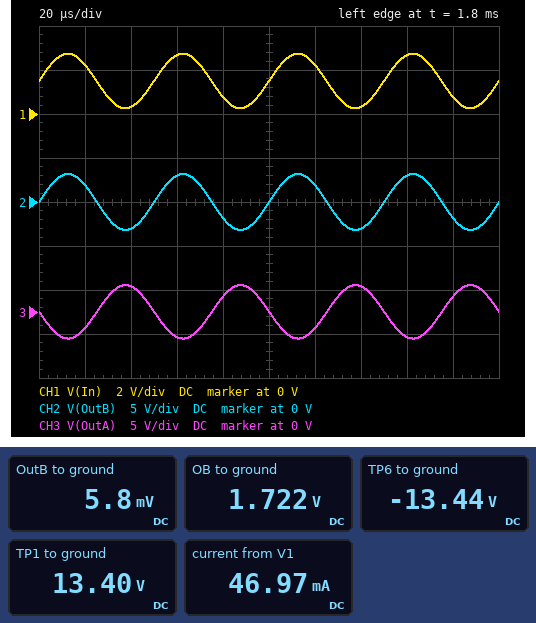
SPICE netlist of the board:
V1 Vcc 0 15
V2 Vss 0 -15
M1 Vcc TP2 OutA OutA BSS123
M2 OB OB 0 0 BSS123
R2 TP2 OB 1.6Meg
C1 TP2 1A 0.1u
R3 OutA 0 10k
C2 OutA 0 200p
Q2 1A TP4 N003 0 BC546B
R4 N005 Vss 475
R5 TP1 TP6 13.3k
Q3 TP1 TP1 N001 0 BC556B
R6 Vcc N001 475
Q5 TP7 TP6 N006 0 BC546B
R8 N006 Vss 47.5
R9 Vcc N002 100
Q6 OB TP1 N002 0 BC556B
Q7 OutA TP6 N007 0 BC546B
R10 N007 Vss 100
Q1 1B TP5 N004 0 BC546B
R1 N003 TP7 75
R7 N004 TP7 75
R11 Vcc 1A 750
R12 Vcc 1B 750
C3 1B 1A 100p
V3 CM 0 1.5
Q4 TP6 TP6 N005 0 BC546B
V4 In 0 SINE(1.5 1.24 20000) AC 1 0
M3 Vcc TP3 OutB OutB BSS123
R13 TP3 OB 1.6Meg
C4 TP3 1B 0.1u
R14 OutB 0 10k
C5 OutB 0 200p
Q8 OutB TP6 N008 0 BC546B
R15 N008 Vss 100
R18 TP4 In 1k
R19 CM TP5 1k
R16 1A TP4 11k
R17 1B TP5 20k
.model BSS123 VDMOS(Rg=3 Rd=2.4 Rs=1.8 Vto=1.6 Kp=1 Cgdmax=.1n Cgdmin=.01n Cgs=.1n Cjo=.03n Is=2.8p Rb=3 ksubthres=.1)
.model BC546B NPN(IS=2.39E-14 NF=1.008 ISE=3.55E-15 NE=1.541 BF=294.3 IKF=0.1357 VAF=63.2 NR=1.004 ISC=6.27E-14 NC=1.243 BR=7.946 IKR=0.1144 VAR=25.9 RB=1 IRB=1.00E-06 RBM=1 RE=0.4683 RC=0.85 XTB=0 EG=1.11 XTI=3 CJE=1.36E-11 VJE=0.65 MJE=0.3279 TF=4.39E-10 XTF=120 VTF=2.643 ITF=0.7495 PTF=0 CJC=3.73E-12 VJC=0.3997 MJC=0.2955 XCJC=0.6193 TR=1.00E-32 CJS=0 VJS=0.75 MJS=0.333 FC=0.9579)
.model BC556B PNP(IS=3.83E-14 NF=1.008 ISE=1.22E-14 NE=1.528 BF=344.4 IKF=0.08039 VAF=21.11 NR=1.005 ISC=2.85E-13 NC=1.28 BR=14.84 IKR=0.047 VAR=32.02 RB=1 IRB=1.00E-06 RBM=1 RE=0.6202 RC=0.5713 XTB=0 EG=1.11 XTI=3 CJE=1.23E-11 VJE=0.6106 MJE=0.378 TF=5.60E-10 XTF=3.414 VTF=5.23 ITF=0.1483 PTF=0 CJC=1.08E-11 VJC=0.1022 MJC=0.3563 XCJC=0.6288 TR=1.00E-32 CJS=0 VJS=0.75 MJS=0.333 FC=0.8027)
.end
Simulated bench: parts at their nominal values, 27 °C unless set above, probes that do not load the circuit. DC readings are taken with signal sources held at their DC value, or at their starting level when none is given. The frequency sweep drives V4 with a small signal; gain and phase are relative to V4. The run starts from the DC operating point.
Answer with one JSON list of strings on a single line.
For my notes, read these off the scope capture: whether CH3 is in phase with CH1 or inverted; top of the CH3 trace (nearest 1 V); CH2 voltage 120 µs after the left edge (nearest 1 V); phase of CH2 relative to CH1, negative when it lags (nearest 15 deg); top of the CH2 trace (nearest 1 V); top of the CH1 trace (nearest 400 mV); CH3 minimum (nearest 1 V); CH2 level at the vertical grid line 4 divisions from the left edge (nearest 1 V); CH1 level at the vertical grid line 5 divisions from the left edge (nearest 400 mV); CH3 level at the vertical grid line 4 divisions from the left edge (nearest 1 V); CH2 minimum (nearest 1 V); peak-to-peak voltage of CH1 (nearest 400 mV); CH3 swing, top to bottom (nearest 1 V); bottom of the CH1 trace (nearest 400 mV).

["inverted", "3 V", "2 V", "0 deg", "3 V", "2.8 V", "-3 V", "-2 V", "1.6 V", "2 V", "-3 V", "2.4 V", "6 V", "400 mV"]
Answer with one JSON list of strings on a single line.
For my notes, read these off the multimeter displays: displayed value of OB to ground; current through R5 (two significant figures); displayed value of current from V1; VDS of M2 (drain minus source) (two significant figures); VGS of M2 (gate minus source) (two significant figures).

["1.722 V", "2.0 mA", "46.97 mA", "1.7 V", "1.7 V"]
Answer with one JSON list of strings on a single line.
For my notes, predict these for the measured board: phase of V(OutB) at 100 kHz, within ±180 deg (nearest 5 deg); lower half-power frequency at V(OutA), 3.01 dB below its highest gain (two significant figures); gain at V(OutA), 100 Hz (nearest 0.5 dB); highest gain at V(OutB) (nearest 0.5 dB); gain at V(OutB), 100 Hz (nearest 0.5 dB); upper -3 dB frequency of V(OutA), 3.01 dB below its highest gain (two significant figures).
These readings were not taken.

["-5 deg", "990 mHz", "8.0 dB", "8.0 dB", "8.0 dB", "1.5 MHz"]
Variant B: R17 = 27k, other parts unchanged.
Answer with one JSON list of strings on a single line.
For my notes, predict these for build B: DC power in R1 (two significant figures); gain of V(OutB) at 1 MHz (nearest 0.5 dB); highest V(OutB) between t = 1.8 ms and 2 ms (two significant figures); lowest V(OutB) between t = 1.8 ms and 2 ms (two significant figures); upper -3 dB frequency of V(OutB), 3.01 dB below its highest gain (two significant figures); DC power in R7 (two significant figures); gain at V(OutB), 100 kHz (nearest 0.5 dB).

["7.6 mW", "7.0 dB", "3.3 V", "-3.3 V", "1.5 MHz", "4.4 mW", "8.5 dB"]
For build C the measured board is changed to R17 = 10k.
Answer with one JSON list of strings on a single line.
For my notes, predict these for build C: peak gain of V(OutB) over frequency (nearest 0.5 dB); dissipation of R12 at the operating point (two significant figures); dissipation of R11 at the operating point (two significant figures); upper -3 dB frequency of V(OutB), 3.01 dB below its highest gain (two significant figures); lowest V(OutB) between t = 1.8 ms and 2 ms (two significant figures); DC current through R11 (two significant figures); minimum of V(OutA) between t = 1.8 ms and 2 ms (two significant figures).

["7.0 dB", "69 mW", "64 mW", "1.8 MHz", "-2.8 V", "9.2 mA", "-2.7 V"]
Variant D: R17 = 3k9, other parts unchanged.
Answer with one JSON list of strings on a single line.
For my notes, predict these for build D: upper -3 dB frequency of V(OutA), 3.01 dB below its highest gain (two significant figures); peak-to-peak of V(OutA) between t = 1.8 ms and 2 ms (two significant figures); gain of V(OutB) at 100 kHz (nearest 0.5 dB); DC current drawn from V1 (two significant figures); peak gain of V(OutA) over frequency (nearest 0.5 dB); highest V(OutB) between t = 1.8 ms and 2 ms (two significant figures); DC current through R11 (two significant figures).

["2.3 MHz", "4.4 V", "4.5 dB", "48 mA", "5.0 dB", "2.1 V", "7.6 mA"]
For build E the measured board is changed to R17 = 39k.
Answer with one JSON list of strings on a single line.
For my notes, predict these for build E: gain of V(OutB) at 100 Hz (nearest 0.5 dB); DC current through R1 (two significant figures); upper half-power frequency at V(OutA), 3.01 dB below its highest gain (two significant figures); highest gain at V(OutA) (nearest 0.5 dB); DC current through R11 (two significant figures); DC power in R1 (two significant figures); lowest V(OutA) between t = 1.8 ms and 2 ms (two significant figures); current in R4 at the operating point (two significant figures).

["9.0 dB", "10 mA", "1.4 MHz", "8.5 dB", "11 mA", "8.1 mW", "-3.2 V", "1.9 mA"]
